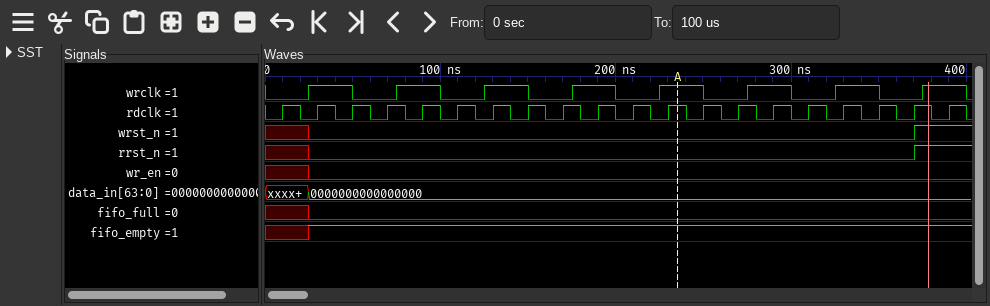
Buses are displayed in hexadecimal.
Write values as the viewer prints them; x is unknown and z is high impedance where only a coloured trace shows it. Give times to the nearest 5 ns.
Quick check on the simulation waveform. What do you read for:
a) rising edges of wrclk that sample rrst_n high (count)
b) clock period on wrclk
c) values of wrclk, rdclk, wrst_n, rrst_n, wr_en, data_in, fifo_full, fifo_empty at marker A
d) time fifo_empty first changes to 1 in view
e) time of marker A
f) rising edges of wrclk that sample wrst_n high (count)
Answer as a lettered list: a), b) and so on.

a) 1
b) 50 ns
c) wrclk=1, rdclk=1, wrst_n=0, rrst_n=0, wr_en=0, data_in=0000000000000000, fifo_full=0, fifo_empty=1
d) 25 ns
e) 235 ns
f) 1
